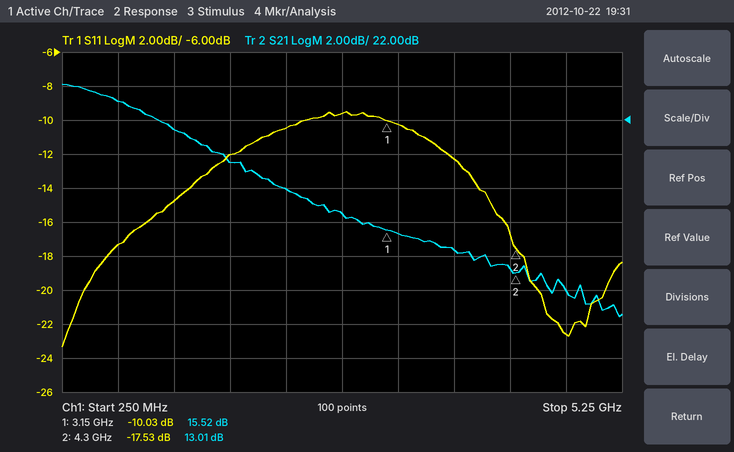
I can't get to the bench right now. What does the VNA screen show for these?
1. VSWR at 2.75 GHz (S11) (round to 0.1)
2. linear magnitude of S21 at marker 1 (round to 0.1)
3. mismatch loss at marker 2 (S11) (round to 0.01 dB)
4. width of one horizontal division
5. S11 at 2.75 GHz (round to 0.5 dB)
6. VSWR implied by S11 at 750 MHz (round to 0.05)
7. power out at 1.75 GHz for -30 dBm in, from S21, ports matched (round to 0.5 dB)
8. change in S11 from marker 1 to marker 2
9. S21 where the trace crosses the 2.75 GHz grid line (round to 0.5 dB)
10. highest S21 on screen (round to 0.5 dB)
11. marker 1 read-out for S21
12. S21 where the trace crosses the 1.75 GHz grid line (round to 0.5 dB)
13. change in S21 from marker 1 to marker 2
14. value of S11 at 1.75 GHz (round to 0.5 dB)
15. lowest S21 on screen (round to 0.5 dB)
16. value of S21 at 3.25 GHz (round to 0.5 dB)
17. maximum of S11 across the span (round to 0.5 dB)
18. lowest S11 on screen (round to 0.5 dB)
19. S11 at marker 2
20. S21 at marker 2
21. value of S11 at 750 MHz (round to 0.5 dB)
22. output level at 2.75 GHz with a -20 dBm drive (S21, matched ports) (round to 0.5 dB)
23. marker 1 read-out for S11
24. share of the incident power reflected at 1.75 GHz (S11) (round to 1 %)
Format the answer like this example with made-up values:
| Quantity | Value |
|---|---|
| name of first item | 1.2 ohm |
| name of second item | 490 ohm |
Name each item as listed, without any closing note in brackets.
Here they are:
| Quantity | Value |
|---|---|
| VSWR at 2.75 GHz (S11) | 2.0 |
| linear magnitude of S21 at marker 1 | 6.0 |
| mismatch loss at marker 2 (S11) | 0.08 dB |
| width of one horizontal division | 500 MHz |
| S11 at 2.75 GHz | -9.5 dB |
| VSWR implied by S11 at 750 MHz | 1.30 |
| power out at 1.75 GHz for -30 dBm in, from S21, ports matched | -10.5 dBm |
| change in S11 from marker 1 to marker 2 | -7.50 dB |
| S21 where the trace crosses the 2.75 GHz grid line | 16.5 dB |
| highest S21 on screen | 24.0 dB |
| marker 1 read-out for S21 | 15.52 dB |
| S21 where the trace crosses the 1.75 GHz grid line | 19.5 dB |
| change in S21 from marker 1 to marker 2 | -2.51 dB |
| value of S11 at 1.75 GHz | -12.0 dB |
| lowest S21 on screen | 10.5 dB |
| value of S21 at 3.25 GHz | 15.5 dB |
| maximum of S11 across the span | -9.5 dB |
| lowest S11 on screen | -23.5 dB |
| S11 at marker 2 | -17.53 dB |
| S21 at marker 2 | 13.01 dB |
| value of S11 at 750 MHz | -17.5 dB |
| output level at 2.75 GHz with a -20 dBm drive (S21, matched ports) | -3.5 dBm |
| marker 1 read-out for S11 | -10.03 dB |
| share of the incident power reflected at 1.75 GHz (S11) | 6 % |
